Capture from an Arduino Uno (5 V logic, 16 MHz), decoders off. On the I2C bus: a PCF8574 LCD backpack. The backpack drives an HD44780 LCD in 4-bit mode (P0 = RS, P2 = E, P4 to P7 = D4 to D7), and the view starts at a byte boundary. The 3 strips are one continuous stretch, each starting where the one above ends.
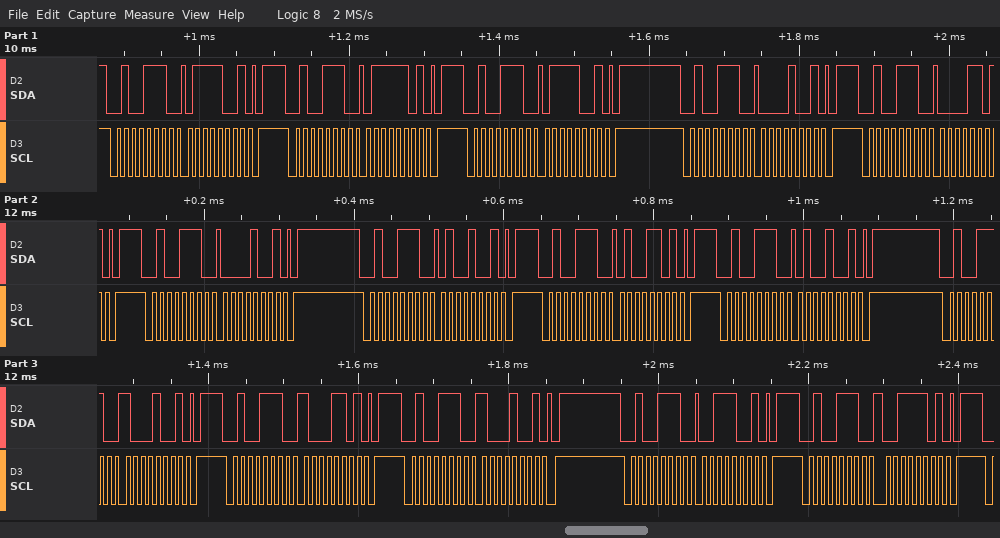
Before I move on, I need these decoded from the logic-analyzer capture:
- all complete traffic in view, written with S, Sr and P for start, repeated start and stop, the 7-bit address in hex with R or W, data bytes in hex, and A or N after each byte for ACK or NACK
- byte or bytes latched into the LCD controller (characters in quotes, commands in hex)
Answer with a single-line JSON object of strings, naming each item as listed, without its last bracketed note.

{"all complete traffic in view, written with S, Sr and P for start, repeated start and stop, the 7-bit address in hex with R or W, data bytes in hex, and A or N after each byte for ACK or NACK": "S 27W A 79 A P S 27W A 7D A P S 27W A 79 A P S 27W A 09 A P S 27W A 0D A P S 27W A 09 A P S 27W A 49 A P S 27W A 4D A P S 27W A 49 A P S 27W A 89 A P S 27W A 8D A P S 27W A 89 A P S 27W A 39 A P S 27W A 3D A P", "byte or bytes latched into the LCD controller": "'p' 'H'"}
